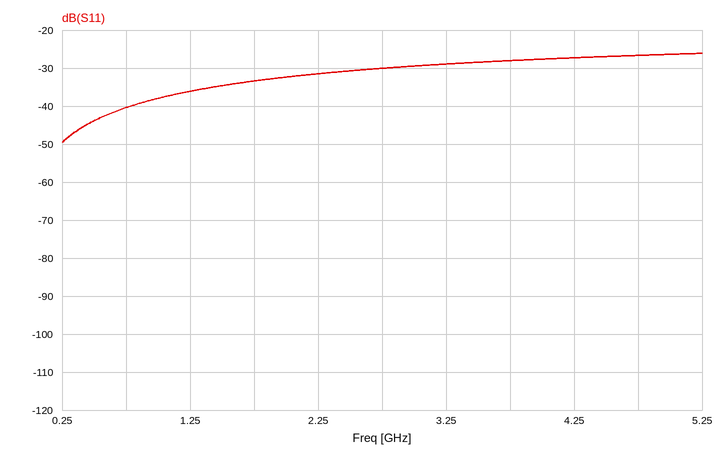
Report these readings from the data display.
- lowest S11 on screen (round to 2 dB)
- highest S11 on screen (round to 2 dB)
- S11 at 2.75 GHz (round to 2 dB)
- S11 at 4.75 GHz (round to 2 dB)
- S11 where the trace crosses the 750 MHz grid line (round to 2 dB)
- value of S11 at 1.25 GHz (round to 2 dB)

-50 dB
-26 dB
-30 dB
-26 dB
-40 dB
-36 dB
